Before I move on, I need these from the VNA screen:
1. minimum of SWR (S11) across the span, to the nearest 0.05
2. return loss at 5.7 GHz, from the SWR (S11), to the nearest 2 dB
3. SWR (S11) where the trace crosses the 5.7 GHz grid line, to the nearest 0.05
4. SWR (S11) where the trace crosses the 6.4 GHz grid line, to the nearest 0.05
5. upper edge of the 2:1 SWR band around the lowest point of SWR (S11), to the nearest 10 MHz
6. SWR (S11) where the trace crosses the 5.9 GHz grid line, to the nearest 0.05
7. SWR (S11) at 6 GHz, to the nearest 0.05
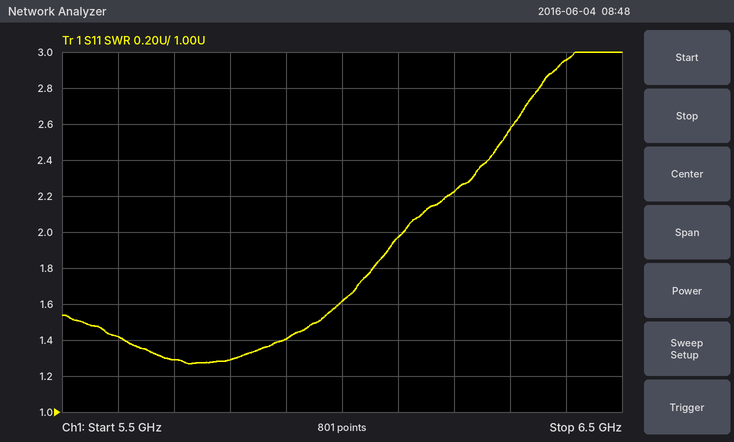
1.25
18 dB
1.30
2.95
6.11 GHz
1.40
1.60
